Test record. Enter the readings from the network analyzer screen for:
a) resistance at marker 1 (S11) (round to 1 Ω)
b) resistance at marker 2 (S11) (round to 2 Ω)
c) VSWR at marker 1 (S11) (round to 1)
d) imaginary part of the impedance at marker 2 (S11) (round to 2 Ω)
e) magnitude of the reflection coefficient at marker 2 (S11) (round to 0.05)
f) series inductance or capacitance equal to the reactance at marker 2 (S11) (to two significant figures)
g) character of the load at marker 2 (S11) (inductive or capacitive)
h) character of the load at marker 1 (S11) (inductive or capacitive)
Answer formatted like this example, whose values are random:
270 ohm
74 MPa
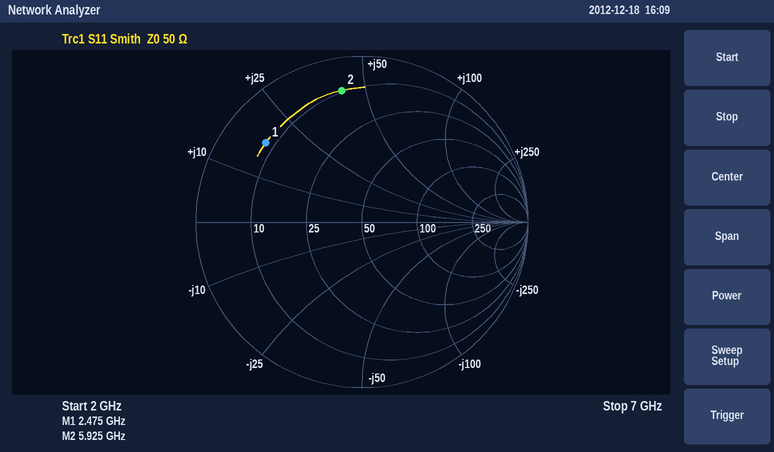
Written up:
8 Ω
10 Ω
7
+42 Ω
0.80
1.1 nH
inductive
inductive
